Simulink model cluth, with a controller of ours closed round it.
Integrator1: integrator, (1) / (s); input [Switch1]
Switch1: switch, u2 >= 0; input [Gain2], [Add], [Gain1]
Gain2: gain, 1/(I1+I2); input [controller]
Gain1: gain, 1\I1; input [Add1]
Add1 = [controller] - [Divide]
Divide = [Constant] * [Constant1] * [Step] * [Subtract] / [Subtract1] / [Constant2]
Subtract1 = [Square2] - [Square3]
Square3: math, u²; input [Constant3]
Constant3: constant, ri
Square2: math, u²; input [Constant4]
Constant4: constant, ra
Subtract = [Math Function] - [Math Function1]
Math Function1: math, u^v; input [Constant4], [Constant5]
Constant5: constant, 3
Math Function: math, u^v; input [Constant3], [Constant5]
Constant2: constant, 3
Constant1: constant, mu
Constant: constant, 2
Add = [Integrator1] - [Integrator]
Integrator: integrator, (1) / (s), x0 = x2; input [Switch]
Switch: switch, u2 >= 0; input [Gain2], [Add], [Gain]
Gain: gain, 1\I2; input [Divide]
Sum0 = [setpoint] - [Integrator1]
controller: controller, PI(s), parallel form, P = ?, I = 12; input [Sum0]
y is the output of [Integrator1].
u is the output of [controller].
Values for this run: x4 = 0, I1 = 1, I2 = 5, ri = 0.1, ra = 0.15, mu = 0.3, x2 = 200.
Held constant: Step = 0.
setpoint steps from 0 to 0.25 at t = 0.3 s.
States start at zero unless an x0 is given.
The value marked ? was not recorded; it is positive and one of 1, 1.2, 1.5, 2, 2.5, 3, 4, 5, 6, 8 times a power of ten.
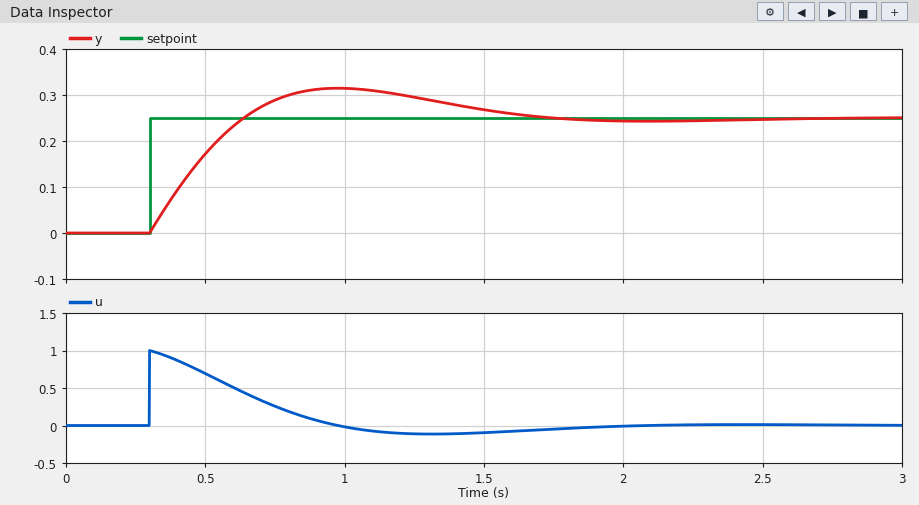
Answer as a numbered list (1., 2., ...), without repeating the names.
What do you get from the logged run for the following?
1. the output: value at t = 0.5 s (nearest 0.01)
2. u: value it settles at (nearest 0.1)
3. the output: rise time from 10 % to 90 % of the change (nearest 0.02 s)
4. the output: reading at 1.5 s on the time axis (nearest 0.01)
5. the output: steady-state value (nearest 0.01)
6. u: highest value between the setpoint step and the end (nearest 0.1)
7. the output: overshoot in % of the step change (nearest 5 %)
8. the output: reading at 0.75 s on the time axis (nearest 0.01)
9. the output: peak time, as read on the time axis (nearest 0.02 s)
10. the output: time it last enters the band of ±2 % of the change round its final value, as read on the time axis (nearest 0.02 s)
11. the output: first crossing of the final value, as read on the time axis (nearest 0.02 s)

1. 0.17
2. 0.0
3. 0.26 s
4. 0.27
5. 0.25
6. 1.0
7. 25 %
8. 0.29
9. 0.98 s
10. 2.36 s
11. 0.64 s
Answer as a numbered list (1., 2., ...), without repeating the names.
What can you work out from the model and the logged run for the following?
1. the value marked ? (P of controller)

1. 4
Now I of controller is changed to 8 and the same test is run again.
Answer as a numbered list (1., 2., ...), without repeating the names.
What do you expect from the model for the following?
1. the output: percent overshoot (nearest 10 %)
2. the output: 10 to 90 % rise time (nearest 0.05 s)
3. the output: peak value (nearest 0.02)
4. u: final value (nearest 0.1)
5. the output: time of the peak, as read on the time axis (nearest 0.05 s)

1. 20 %
2. 0.30 s
3. 0.30
4. 0.0
5. 1.10 s
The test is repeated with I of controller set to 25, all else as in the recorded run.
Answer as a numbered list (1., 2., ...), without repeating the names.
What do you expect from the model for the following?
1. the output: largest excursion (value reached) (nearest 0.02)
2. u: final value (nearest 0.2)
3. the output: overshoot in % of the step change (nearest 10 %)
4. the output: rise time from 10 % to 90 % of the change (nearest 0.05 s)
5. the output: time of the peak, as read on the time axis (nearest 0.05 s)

1. 0.34
2. 0.0
3. 40 %
4. 0.20 s
5. 0.80 s
